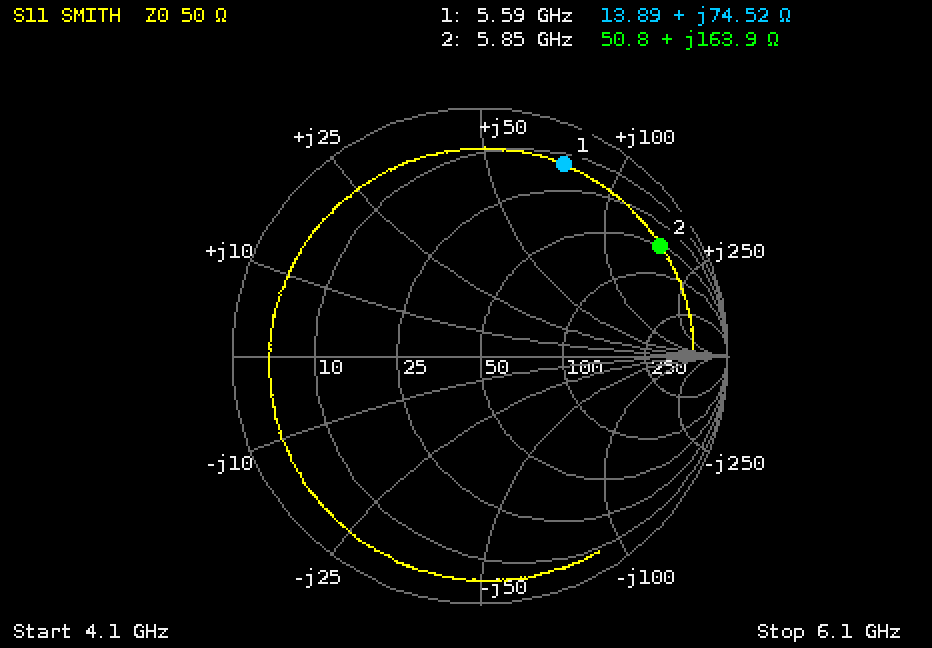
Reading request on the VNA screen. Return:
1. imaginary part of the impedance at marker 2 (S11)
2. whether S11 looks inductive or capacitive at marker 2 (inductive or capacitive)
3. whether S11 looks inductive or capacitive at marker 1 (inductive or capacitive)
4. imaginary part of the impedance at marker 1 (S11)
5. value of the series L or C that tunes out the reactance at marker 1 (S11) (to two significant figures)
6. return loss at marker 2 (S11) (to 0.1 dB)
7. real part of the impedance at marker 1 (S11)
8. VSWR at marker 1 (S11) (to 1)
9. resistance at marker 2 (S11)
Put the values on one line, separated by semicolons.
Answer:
+163.9 Ω; inductive; inductive; +74.52 Ω; 380 fF; 1.4 dB; 13.89 Ω; 12; 50.8 Ω
